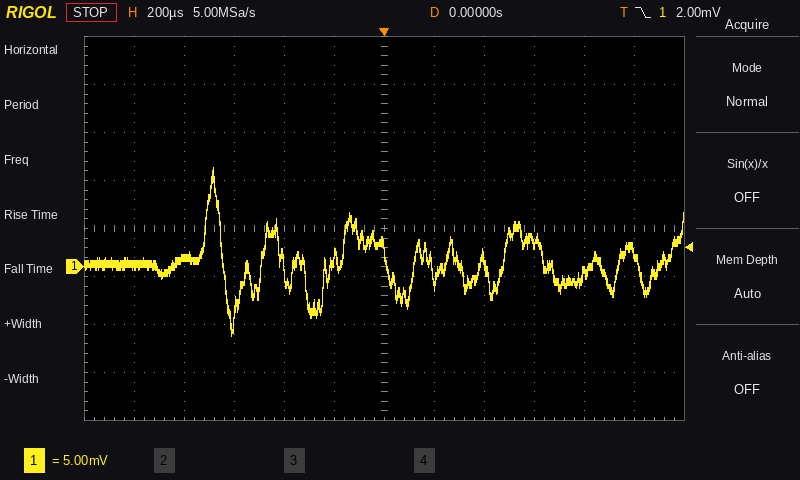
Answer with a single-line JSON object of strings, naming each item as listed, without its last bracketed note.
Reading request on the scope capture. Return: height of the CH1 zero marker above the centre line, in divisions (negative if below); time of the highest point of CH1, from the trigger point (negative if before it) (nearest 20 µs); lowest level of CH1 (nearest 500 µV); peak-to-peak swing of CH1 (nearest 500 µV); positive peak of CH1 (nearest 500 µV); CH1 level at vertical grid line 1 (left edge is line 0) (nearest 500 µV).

{"height of the CH1 zero marker above the centre line, in divisions": "-0.8 div", "time of the highest point of CH1, from the trigger point (negative if before it)": "-680 µs", "lowest level of CH1": "-7.0 mV", "peak-to-peak swing of CH1": "17.5 mV", "positive peak of CH1": "10.5 mV", "CH1 level at vertical grid line 1 (left edge is line 0)": "0.0 mV"}
